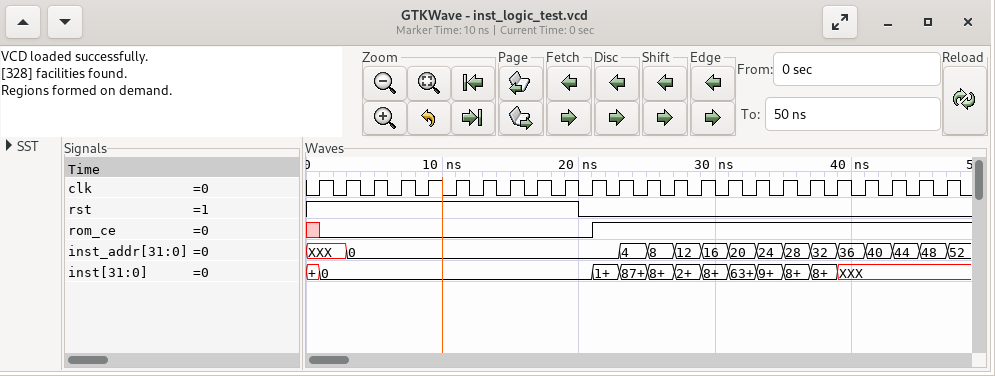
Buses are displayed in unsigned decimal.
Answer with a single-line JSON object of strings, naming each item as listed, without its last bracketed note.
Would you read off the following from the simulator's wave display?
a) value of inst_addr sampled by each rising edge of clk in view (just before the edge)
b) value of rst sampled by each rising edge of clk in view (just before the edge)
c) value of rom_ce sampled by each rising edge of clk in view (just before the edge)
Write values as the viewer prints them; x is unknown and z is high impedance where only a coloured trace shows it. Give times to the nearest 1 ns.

{"value of inst_addr sampled by each rising edge of clk in view": "XXX, XXX, 0, 0, 0, 0, 0, 0, 0, 0, 0, 0, 4, 8, 12, 16, 20, 24, 28, 32, 36, 40, 44, 48", "value of rst sampled by each rising edge of clk in view": "1 1 1 1 1 1 1 1 1 1 0 0 0 0 0 0 0 0 0 0 0 0 0 0", "value of rom_ce sampled by each rising edge of clk in view": "x 0 0 0 0 0 0 0 0 0 0 1 1 1 1 1 1 1 1 1 1 1 1 1"}
